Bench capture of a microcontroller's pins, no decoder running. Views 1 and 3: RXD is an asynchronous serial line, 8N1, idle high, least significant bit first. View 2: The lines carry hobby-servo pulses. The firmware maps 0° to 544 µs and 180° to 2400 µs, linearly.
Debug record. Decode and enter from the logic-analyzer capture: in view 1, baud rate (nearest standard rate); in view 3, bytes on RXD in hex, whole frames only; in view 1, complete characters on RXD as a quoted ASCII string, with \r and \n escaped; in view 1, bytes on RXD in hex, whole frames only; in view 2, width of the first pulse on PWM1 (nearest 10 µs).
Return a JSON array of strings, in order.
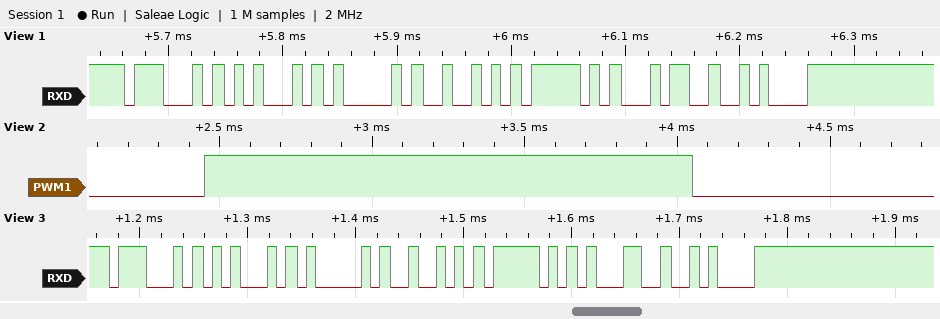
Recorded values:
["115200 baud", "0x47 0x45 0x41 0x52 0x5F 0x31 0x0A", "\"GEAR_4\\n\"", "47 45 41 52 5F 34 0A", "1600 µs"]
